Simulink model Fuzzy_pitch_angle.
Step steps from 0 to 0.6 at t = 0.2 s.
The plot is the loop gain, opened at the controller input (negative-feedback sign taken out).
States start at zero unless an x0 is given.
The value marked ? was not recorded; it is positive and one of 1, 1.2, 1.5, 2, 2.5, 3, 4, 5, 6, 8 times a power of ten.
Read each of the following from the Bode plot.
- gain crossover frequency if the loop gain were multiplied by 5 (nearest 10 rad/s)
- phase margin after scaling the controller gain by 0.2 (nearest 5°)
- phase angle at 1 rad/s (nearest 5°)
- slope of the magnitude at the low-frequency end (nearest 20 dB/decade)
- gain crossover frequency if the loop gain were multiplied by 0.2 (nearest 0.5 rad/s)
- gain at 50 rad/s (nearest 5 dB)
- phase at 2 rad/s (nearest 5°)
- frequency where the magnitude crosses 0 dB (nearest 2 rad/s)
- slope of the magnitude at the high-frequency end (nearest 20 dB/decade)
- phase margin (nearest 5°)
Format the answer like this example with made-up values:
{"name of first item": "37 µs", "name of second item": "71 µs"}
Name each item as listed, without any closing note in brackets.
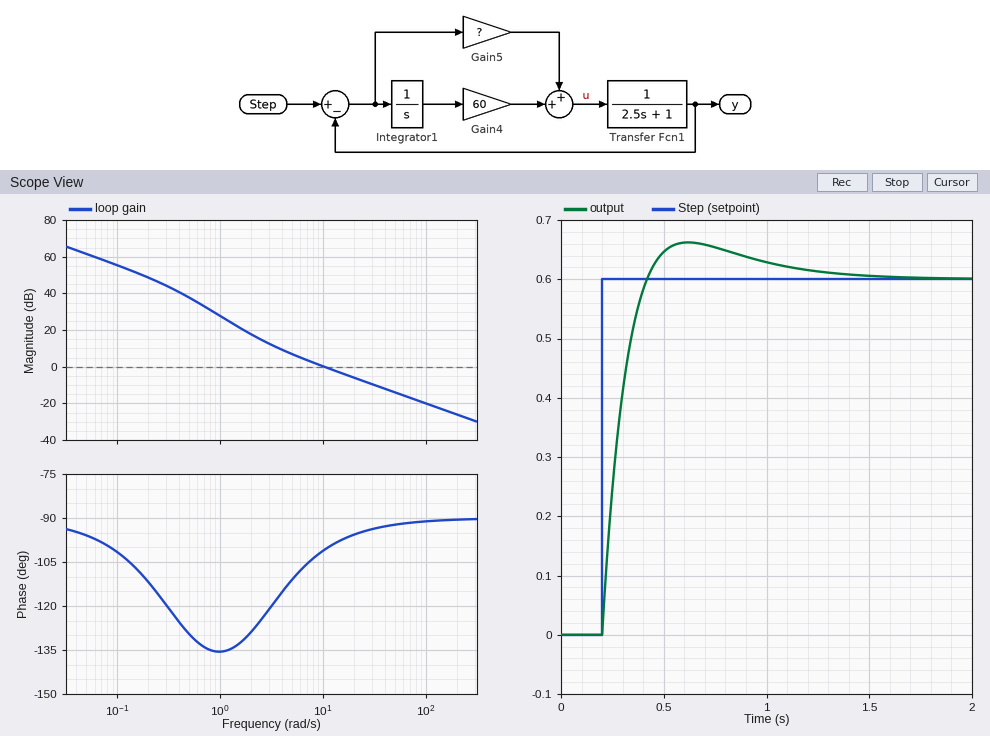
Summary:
{"gain crossover frequency if the loop gain were multiplied by 5": "50 rad/s", "phase margin after scaling the controller gain by 0.2": "55°", "phase angle at 1 rad/s": "-135°", "slope of the magnitude at the low-frequency end": "-20 dB/decade", "gain crossover frequency if the loop gain were multiplied by 0.2": "2.5 rad/s", "gain at 50 rad/s": "-15 dB", "phase at 2 rad/s": "-130°", "frequency where the magnitude crosses 0 dB": "10 rad/s", "slope of the magnitude at the high-frequency end": "-20 dB/decade", "phase margin": "80°"}
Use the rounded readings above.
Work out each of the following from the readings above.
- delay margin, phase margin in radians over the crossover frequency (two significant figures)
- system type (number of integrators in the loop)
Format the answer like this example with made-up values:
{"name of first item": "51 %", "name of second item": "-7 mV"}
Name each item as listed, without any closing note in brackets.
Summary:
{"delay margin, phase margin in radians over the crossover frequency": "0.14 s", "system type": "1"}
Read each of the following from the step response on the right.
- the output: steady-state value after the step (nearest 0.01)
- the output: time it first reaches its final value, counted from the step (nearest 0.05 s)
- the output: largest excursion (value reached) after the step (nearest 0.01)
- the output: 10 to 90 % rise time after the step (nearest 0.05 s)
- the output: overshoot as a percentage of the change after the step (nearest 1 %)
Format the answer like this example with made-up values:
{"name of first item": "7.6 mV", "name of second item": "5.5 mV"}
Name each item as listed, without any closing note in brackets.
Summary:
{"the output: steady-state value after the step": "0.60", "the output: time it first reaches its final value, counted from the step": "0.20 s", "the output: largest excursion (value reached) after the step": "0.66", "the output: 10 to 90 % rise time after the step": "0.15 s", "the output: overshoot as a percentage of the change after the step": "10 %"}
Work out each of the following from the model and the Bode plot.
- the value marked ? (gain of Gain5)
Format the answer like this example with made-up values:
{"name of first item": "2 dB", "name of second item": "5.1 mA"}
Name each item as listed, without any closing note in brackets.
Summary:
{"the value marked ?": "25"}
